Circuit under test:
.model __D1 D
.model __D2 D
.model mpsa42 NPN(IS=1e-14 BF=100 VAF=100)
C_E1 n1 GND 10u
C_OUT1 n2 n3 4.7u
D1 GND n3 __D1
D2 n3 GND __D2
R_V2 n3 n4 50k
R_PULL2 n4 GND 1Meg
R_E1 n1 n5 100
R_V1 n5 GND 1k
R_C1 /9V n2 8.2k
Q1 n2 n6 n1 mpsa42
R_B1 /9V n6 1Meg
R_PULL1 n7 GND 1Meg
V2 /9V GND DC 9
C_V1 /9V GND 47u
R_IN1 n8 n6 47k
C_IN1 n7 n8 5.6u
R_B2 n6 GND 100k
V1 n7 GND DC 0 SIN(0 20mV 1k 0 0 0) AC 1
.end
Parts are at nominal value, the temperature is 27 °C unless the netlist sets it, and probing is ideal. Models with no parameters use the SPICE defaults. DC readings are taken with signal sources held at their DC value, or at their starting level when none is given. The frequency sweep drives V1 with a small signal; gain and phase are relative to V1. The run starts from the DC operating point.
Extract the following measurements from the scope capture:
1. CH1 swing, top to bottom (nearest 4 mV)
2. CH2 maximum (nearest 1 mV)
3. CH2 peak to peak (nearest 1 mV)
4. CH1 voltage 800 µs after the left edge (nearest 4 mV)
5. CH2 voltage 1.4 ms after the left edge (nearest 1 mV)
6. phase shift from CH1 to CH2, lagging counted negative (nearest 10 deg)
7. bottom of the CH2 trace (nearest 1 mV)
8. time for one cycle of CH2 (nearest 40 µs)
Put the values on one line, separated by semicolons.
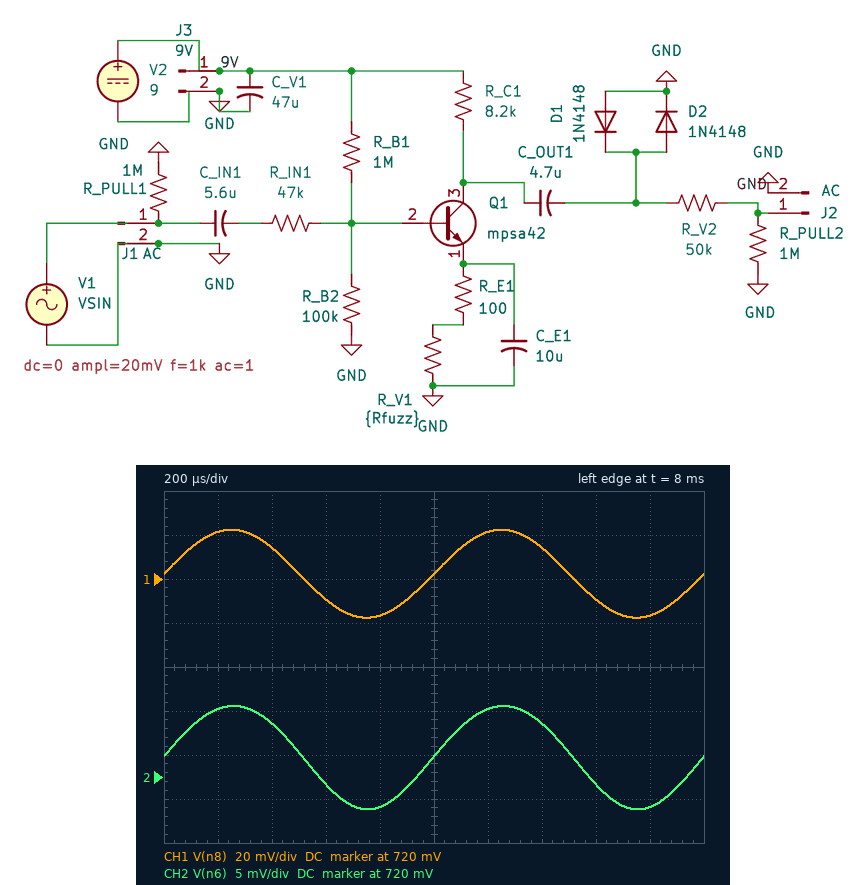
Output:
40 mV; 728 mV; 12 mV; 704 mV; 726 mV; 0 deg; 716 mV; 1.00 ms
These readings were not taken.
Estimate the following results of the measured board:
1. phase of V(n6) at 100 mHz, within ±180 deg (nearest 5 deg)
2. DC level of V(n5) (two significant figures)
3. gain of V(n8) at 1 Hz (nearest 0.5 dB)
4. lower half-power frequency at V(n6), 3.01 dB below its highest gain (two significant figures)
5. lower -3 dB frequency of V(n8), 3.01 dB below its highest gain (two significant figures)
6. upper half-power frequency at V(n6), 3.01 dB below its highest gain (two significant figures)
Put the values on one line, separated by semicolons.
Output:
70 deg; 110 mV; -0.5 dB; 270 mHz; 280 mHz; 72 Hz
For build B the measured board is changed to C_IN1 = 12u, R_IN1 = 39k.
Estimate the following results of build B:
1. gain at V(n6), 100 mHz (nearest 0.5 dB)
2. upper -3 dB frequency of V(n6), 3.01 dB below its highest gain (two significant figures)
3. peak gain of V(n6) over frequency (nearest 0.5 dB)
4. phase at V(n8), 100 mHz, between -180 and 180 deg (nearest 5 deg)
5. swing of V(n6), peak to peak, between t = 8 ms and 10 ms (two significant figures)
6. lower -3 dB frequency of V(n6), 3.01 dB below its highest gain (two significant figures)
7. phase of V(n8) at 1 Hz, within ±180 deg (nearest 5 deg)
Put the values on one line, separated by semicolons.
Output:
-9.5 dB; 80 Hz; -4.5 dB; 55 deg; 13 mV; 140 mHz; 10 deg
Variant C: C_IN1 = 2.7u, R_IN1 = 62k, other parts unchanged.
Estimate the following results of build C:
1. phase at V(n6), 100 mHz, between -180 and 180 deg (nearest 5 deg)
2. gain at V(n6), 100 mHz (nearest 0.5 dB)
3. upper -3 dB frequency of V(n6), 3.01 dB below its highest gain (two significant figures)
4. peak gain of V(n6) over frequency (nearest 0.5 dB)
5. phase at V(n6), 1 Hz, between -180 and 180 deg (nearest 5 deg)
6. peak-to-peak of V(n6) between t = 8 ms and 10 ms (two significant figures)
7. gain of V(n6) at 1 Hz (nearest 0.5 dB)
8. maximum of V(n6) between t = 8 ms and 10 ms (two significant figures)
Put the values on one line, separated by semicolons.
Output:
80 deg; -20.5 dB; 63 Hz; -6.5 dB; 25 deg; 9.6 mV; -7.5 dB; 730 mV
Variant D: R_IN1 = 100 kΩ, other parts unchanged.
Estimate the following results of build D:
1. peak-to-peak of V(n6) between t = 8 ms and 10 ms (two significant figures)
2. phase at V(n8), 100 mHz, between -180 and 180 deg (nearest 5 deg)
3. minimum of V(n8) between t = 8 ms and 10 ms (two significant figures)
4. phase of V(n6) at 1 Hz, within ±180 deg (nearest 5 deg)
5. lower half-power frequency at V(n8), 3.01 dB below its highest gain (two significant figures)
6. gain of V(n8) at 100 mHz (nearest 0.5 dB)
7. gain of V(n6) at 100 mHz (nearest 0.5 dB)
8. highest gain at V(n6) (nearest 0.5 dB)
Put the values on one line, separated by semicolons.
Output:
6.5 mV; 60 deg; 700 mV; 10 deg; 180 mHz; -6.5 dB; -15.5 dB; -9.0 dB
